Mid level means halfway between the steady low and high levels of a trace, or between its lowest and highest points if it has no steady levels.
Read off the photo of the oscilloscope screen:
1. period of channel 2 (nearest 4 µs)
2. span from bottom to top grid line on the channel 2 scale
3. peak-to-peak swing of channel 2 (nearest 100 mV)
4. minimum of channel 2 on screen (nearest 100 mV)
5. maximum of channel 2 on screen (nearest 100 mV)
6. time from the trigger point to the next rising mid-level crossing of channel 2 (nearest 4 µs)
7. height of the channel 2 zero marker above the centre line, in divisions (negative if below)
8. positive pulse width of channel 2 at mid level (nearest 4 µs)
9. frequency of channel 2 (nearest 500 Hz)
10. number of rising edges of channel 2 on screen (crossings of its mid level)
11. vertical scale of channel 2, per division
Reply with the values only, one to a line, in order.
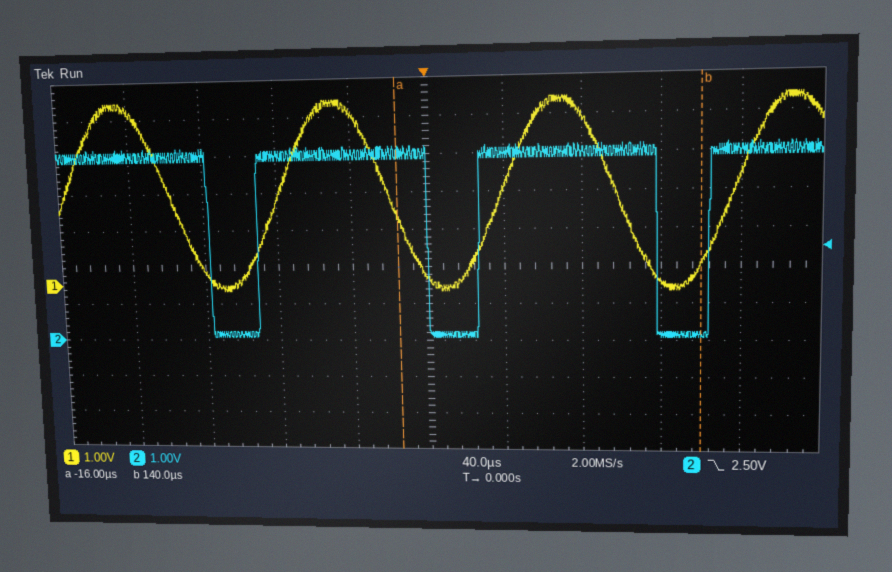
116 µs
10 V
5.1 V
100 mV
5.2 V
28 µs
-2.0 div
92 µs
8.5 kHz
3
1 V
